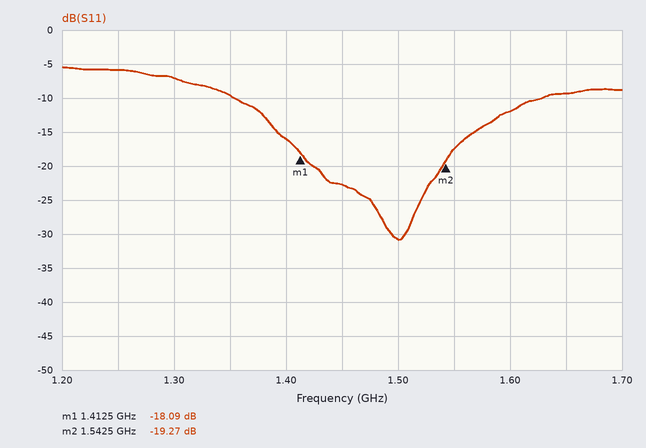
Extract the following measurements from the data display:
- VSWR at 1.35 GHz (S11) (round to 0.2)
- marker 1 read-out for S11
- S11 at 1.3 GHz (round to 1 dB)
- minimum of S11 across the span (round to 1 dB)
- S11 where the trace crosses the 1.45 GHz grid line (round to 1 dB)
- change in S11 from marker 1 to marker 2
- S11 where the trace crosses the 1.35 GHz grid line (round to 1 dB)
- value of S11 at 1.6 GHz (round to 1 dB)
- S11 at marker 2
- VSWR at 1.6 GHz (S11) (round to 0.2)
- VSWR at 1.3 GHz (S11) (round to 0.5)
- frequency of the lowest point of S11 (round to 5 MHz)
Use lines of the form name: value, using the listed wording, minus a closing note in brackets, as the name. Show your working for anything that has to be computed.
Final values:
VSWR at 1.35 GHz (S11): |Γ| = 10^(-10/20) = 0.3162; VSWR = (1 + 0.3162)/(1 − 0.3162) ≈ 1.92, so 2.0 to the nearest 0.2
marker 1 read-out for S11: -18.09 dB
S11 at 1.3 GHz: -7 dB
minimum of S11 across the span: -31 dB
S11 where the trace crosses the 1.45 GHz grid line: -23 dB
change in S11 from marker 1 to marker 2: -19.27 − (-18.09) = -1.18 dB
S11 where the trace crosses the 1.35 GHz grid line: -10 dB
value of S11 at 1.6 GHz: -12 dB
S11 at marker 2: -19.27 dB
VSWR at 1.6 GHz (S11): |Γ| = 10^(-12/20) = 0.2512; VSWR = (1 + 0.2512)/(1 − 0.2512) ≈ 1.67, so 1.6 to the nearest 0.2
VSWR at 1.3 GHz (S11): |Γ| = 10^(-7/20) = 0.4467; VSWR = (1 + 0.4467)/(1 − 0.4467) ≈ 2.61, so 2.5 to the nearest 0.5
frequency of the lowest point of S11: 1.500 GHz
